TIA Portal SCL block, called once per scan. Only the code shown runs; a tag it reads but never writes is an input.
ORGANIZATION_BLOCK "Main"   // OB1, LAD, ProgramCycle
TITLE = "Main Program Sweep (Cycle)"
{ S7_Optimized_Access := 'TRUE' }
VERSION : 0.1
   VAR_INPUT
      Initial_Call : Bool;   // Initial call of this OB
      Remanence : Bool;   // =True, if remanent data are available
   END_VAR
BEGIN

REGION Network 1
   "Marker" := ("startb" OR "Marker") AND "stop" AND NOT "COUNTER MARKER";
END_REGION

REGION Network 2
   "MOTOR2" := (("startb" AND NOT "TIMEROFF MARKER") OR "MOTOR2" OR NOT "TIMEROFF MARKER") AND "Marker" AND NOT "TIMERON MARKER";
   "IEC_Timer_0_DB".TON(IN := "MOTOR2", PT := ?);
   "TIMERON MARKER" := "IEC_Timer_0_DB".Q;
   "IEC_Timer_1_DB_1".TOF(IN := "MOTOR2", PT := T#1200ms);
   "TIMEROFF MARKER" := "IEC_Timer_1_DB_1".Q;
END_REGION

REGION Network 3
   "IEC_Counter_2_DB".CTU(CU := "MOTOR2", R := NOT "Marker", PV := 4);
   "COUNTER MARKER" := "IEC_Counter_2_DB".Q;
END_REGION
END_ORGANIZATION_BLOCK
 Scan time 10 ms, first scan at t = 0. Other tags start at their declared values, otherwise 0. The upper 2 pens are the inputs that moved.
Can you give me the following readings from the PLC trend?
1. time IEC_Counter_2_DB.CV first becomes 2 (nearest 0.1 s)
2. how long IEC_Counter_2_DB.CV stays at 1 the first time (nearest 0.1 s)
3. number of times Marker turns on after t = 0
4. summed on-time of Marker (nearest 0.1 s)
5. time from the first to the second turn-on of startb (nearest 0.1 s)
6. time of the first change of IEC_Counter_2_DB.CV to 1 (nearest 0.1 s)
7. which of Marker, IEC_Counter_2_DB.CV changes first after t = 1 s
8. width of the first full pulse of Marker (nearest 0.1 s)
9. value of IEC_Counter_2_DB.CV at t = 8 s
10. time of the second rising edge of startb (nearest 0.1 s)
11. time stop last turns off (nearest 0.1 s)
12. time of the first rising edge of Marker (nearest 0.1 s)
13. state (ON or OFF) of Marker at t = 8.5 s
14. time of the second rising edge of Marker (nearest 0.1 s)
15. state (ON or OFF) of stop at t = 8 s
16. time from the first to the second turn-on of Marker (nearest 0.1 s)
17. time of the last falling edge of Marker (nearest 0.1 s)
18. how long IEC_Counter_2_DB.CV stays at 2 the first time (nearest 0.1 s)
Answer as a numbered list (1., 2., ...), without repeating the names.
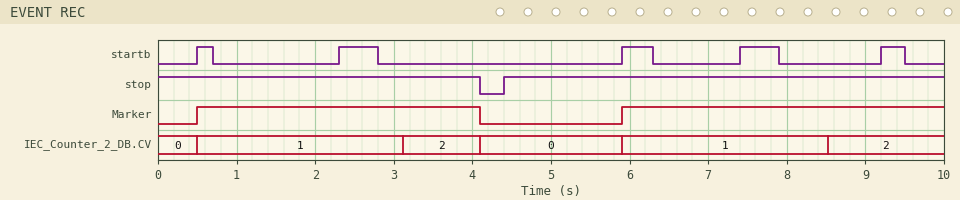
1. 3.1 s
2. 2.6 s
3. 2
4. 7.7 s
5. 1.8 s
6. 0.5 s
7. IEC_Counter_2_DB.CV
8. 3.6 s
9. 1
10. 2.3 s
11. 4.1 s
12. 0.5 s
13. ON
14. 5.9 s
15. ON
16. 5.4 s
17. 4.1 s
18. 1.0 s
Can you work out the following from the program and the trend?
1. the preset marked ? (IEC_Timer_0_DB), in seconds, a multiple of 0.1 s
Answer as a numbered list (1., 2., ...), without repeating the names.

1. 1.4 s
